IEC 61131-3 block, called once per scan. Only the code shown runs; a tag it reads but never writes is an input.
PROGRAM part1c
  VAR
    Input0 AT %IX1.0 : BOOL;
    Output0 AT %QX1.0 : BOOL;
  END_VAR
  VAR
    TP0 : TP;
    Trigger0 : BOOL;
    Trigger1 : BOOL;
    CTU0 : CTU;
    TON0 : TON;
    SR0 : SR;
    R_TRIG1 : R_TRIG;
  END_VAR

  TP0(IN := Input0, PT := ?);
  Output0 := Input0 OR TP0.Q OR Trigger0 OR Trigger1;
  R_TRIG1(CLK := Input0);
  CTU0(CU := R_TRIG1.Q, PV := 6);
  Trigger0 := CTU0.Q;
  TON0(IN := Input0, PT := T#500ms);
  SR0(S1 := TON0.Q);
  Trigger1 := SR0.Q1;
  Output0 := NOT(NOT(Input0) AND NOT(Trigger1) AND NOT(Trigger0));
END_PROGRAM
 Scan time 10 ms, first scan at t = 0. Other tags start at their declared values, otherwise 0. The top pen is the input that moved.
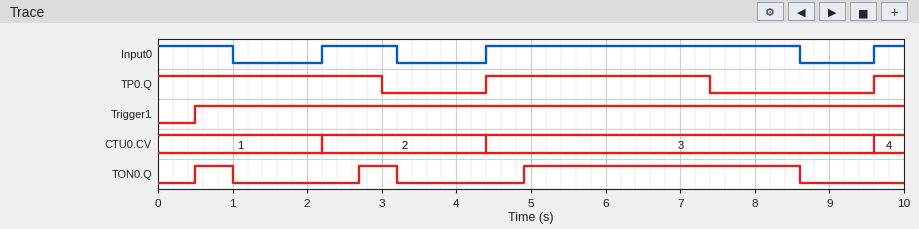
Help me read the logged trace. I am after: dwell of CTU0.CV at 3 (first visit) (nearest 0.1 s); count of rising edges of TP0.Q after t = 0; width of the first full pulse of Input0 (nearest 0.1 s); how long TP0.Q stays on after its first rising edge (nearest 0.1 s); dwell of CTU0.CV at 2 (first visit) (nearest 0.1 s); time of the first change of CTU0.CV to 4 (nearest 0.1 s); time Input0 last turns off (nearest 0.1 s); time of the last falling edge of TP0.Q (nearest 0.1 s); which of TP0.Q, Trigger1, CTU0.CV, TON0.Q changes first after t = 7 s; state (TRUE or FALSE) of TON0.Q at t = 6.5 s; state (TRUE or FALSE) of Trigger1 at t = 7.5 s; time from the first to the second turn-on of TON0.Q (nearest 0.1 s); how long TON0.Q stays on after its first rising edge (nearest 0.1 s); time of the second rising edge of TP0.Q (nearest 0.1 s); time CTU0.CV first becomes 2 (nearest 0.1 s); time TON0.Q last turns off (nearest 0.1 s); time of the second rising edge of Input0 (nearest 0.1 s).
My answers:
5.2 s
2
1.0 s
3.0 s
2.2 s
9.6 s
8.6 s
7.4 s
TP0.Q
TRUE
TRUE
2.2 s
0.5 s
9.6 s
2.2 s
8.6 s
4.4 s
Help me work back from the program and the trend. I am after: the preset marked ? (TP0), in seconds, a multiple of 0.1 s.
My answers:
3.0 s
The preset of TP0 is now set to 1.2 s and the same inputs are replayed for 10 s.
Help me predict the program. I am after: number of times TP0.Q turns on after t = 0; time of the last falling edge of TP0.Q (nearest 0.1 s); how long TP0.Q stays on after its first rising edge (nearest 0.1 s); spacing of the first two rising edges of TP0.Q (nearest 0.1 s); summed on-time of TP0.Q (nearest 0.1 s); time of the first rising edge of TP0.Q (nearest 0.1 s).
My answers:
3
5.6 s
1.2 s
2.2 s
4.0 s
2.2 s
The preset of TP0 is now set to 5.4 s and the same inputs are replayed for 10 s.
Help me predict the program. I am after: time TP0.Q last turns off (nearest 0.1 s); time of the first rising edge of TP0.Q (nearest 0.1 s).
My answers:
5.4 s
9.6 s
